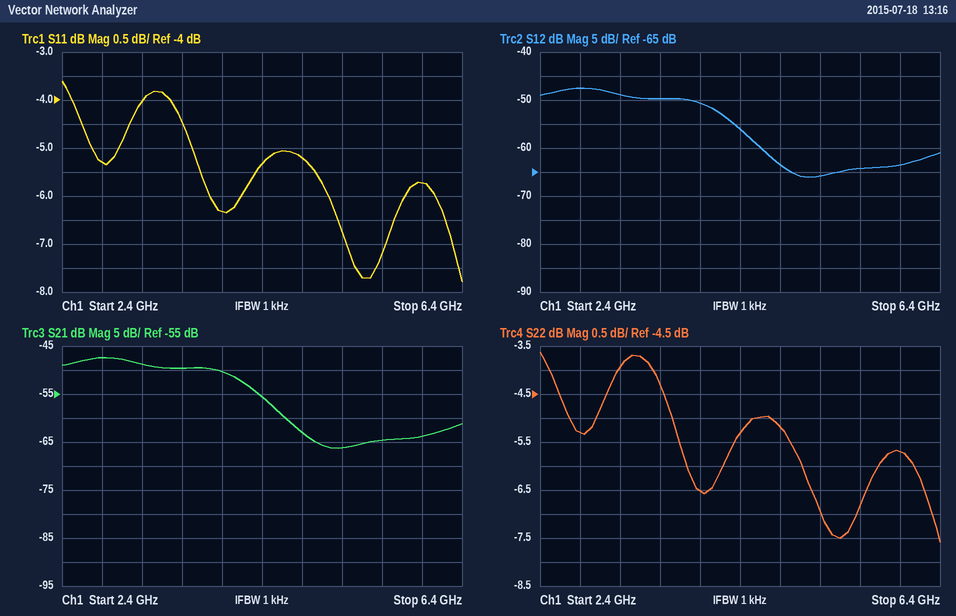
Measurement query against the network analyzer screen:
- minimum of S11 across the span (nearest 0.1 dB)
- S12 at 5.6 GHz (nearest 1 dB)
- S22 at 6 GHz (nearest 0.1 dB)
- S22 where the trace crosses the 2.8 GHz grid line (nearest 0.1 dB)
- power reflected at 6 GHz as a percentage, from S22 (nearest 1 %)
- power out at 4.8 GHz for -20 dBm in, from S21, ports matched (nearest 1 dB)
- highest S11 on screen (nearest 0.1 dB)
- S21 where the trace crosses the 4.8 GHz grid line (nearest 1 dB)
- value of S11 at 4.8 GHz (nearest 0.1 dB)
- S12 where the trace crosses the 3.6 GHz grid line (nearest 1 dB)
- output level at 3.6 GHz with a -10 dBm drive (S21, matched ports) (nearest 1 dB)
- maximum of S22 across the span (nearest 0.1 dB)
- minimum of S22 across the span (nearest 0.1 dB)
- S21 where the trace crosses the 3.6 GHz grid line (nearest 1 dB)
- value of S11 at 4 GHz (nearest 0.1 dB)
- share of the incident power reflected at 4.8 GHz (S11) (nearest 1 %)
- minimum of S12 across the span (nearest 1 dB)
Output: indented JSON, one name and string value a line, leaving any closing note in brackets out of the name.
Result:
{
  "minimum of S11 across the span": "-7.8 dB",
  "S12 at 5.6 GHz": "-64 dB",
  "S22 at 6 GHz": "-5.7 dB",
  "S22 where the trace crosses the 2.8 GHz grid line": "-5.3 dB",
  "power reflected at 6 GHz as a percentage, from S22": "27 %",
  "power out at 4.8 GHz for -20 dBm in, from S21, ports matched": "-83 dBm",
  "highest S11 on screen": "-3.6 dB",
  "S21 where the trace crosses the 4.8 GHz grid line": "-63 dB",
  "value of S11 at 4.8 GHz": "-5.2 dB",
  "S12 where the trace crosses the 3.6 GHz grid line": "-50 dB",
  "output level at 3.6 GHz with a -10 dBm drive (S21, matched ports)": "-60 dBm",
  "maximum of S22 across the span": "-3.6 dB",
  "minimum of S22 across the span": "-7.6 dB",
  "S21 where the trace crosses the 3.6 GHz grid line": "-50 dB",
  "value of S11 at 4 GHz": "-6.3 dB",
  "share of the incident power reflected at 4.8 GHz (S11)": "30 %",
  "minimum of S12 across the span": "-66 dB"
}
